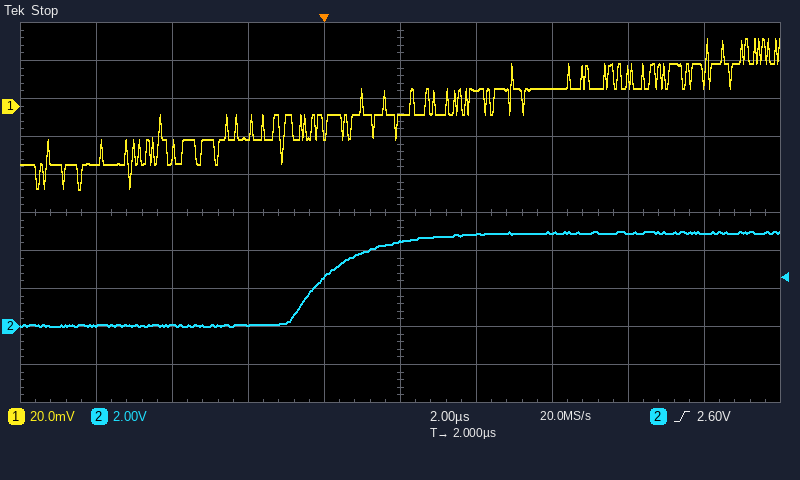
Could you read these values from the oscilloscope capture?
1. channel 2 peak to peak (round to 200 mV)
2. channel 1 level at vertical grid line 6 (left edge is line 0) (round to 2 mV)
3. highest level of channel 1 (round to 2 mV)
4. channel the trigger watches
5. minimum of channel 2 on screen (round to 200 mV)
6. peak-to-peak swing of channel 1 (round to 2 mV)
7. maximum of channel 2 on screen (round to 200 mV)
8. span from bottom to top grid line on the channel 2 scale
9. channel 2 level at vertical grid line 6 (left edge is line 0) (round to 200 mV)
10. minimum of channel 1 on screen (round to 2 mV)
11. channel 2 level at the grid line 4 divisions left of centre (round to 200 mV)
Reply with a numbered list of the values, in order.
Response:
1. 5.0 V
2. 8 mV
3. 36 mV
4. channel 2
5. 0.0 V
6. 80 mV
7. 5.0 V
8. 20 V
9. 4.8 V
10. -44 mV
11. 0.0 V
